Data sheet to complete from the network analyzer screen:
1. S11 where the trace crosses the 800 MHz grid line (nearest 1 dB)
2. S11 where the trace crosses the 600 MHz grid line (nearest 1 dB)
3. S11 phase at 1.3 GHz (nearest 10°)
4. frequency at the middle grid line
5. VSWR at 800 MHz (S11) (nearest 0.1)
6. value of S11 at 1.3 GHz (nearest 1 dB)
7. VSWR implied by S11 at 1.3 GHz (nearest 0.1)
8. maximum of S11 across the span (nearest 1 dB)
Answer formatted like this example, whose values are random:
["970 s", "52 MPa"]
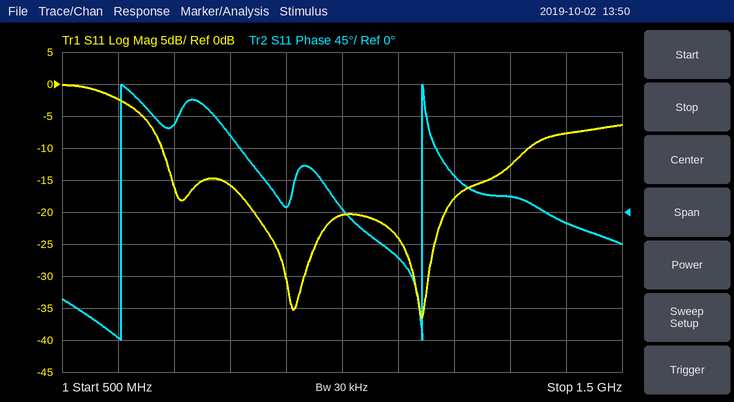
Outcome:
["-16 dB", "-2 dB", "20°", "1 GHz", "1.4", "-13 dB", "1.6", "0 dB"]
